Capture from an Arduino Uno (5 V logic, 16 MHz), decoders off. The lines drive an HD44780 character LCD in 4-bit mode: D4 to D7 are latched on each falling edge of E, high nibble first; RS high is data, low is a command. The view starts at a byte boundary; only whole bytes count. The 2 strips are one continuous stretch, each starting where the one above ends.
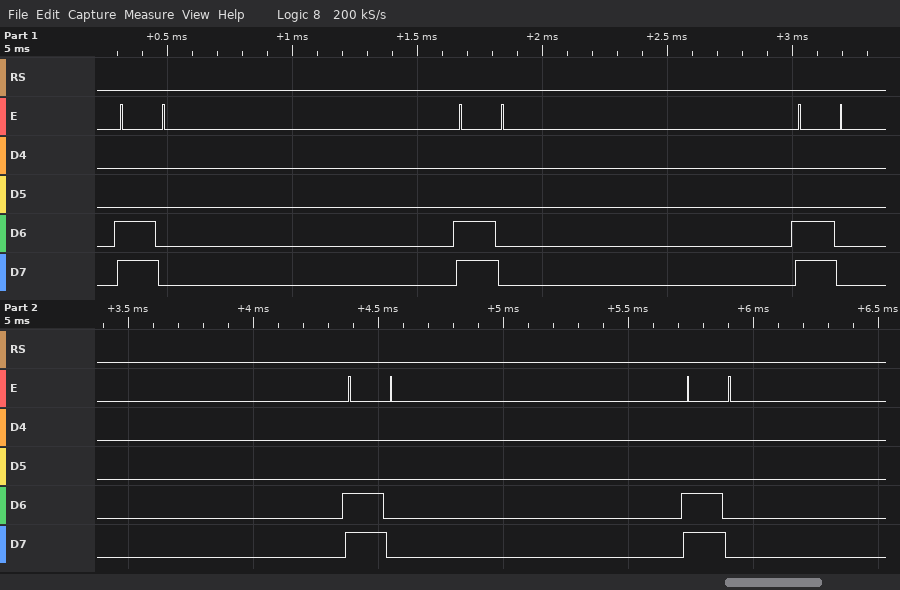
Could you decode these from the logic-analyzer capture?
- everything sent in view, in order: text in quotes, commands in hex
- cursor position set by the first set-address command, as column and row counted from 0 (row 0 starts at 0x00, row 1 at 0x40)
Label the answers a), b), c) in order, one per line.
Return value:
a) 0xC0 0xC0 0xC0 0xC0 0xC0
b) column 0, row 1
